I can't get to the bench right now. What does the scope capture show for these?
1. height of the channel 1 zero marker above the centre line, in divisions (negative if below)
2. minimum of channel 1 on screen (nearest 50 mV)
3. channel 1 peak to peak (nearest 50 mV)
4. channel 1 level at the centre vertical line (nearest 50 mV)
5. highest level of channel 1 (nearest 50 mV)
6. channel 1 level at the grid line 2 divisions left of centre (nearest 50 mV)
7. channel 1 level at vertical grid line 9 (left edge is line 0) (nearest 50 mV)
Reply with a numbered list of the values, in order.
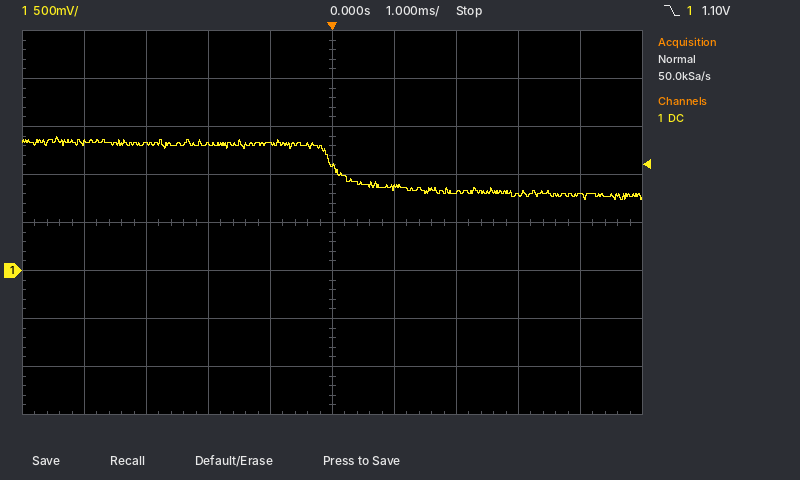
1. -1.0 div
2. 750 mV
3. 650 mV
4. 1.10 V
5. 1.40 V
6. 1.30 V
7. 800 mV
